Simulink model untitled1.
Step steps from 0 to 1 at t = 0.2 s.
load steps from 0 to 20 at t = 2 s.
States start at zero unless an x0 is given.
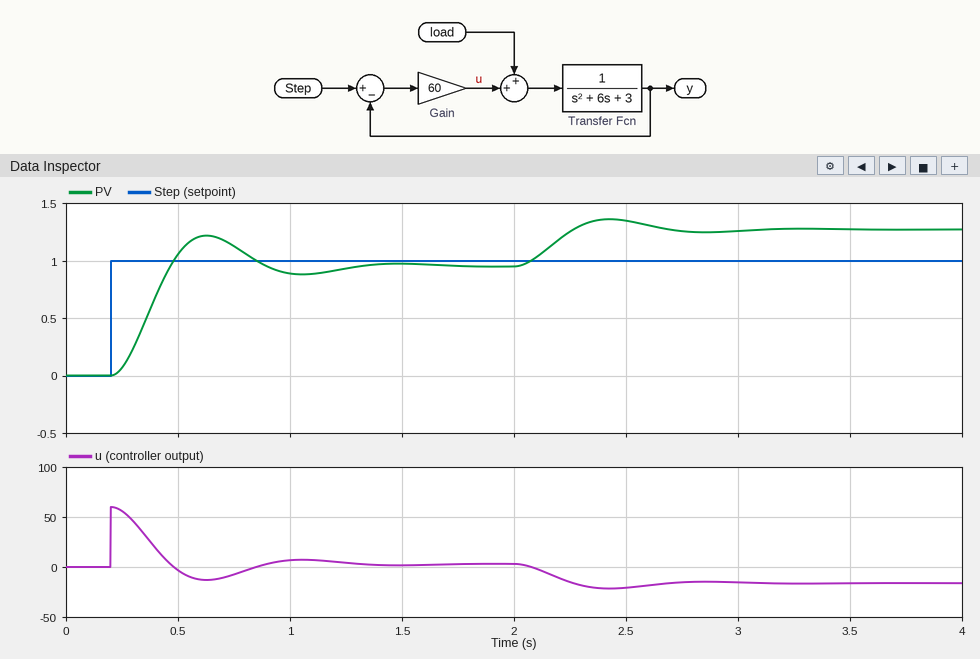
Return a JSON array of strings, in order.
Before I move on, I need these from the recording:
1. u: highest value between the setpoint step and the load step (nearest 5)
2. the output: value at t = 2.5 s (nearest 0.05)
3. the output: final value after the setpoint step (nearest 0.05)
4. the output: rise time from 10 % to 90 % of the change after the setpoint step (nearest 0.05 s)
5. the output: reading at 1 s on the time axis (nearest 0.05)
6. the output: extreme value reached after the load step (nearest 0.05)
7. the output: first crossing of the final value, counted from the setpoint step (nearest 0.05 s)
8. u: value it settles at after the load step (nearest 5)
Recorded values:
["60", "1.35", "0.95", "0.20 s", "0.90", "1.35", "0.25 s", "-15"]
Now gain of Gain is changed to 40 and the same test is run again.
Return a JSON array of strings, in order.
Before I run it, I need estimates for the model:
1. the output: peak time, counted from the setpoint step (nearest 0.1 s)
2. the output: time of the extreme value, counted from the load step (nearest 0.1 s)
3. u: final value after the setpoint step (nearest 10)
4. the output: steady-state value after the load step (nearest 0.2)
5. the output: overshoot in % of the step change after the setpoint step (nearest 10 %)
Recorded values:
["0.5 s", "0.5 s", "0", "1.4", "20 %"]
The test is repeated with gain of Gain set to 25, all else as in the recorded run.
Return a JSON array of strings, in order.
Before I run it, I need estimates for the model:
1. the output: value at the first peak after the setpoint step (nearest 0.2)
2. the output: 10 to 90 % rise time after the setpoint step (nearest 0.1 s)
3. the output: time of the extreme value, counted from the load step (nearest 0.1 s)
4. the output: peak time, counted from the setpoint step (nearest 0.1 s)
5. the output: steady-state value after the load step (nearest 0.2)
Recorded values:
["1.0", "0.3 s", "0.7 s", "0.7 s", "1.6"]
